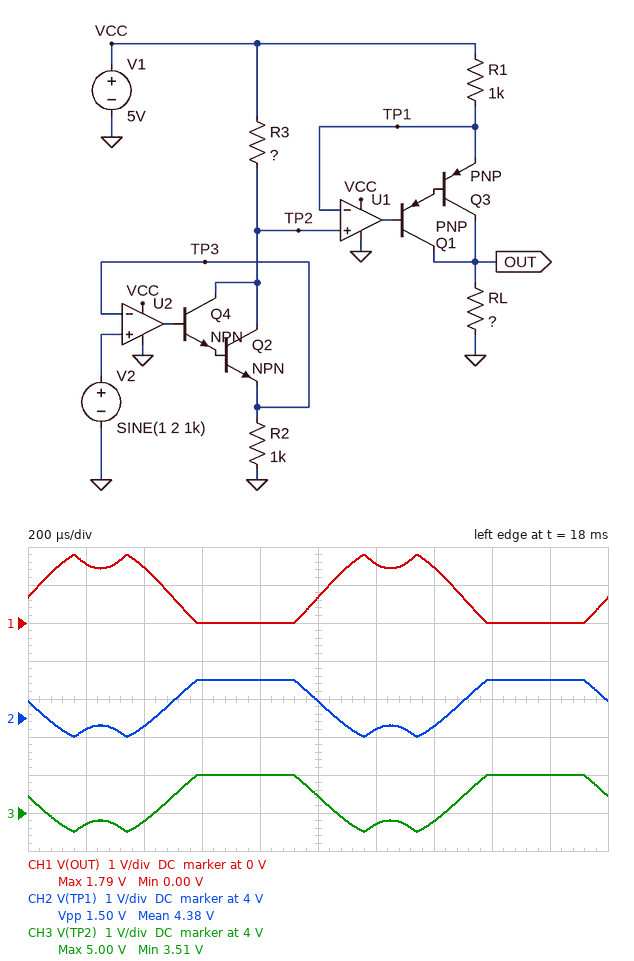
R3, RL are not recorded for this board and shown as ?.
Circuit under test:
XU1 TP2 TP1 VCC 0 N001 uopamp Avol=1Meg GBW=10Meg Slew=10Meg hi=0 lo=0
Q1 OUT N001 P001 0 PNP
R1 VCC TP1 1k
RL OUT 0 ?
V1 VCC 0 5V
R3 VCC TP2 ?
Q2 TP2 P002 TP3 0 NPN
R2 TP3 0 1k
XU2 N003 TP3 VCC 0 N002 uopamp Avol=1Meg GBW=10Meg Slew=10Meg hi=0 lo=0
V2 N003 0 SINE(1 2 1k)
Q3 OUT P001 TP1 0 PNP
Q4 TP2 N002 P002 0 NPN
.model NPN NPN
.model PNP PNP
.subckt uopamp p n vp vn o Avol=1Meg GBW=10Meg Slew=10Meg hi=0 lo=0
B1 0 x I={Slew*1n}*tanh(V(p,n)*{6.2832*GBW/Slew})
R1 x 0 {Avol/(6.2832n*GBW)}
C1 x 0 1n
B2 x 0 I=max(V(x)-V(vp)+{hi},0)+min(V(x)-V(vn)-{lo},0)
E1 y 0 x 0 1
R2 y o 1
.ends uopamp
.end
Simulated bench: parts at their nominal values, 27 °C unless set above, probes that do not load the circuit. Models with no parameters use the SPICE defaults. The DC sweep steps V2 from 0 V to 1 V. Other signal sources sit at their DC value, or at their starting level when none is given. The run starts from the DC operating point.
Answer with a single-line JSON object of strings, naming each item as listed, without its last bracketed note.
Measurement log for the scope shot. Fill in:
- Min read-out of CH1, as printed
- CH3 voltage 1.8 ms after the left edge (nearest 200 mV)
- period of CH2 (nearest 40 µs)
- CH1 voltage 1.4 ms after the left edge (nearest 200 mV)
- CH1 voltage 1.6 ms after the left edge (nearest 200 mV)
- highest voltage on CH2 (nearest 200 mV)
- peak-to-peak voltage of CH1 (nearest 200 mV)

{"Min read-out of CH1, as printed": "0.00 V", "CH3 voltage 1.8 ms after the left edge": "5.0 V", "period of CH2": "1.00 ms", "CH1 voltage 1.4 ms after the left edge": "1.4 V", "CH1 voltage 1.6 ms after the left edge": "0 V", "highest voltage on CH2": "5.0 V", "peak-to-peak voltage of CH1": "1.8 V"}
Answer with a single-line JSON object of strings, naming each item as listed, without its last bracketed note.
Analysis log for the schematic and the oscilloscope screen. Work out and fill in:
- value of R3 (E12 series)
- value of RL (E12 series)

{"value of R3": "560 Ω", "value of RL": "1.2 kΩ"}
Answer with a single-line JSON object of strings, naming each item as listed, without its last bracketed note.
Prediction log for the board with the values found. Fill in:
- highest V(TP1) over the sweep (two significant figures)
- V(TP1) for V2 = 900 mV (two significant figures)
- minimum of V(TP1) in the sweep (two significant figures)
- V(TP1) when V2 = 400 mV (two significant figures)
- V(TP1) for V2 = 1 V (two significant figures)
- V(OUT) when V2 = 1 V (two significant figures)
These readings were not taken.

{"highest V(TP1) over the sweep": "5.0 V", "V(TP1) for V2 = 900 mV": "4.5 V", "minimum of V(TP1) in the sweep": "4.4 V", "V(TP1) when V2 = 400 mV": "4.8 V", "V(TP1) for V2 = 1 V": "4.4 V", "V(OUT) when V2 = 1 V": "670 mV"}
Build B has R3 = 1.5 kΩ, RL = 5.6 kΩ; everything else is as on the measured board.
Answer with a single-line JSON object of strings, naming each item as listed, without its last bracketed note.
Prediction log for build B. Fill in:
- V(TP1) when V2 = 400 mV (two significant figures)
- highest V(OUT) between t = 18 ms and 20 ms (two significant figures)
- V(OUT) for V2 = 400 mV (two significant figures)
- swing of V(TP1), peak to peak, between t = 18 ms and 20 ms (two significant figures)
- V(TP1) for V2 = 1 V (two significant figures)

{"V(TP1) when V2 = 400 mV": "4.4 V", "highest V(OUT) between t = 18 ms and 20 ms": "3.6 V", "V(OUT) for V2 = 400 mV": "3.4 V", "swing of V(TP1), peak to peak, between t = 18 ms and 20 ms": "2.5 V", "V(TP1) for V2 = 1 V": "3.5 V"}
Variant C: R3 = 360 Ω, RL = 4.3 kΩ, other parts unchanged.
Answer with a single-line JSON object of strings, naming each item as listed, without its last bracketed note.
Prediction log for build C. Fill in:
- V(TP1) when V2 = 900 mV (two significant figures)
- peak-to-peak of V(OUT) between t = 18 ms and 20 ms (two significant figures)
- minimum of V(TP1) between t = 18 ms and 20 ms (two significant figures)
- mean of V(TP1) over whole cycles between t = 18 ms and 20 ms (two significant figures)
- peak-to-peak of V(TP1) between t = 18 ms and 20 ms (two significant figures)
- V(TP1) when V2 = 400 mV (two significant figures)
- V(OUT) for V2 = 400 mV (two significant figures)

{"V(TP1) when V2 = 900 mV": "4.7 V", "peak-to-peak of V(OUT) between t = 18 ms and 20 ms": "3.4 V", "minimum of V(TP1) between t = 18 ms and 20 ms": "3.9 V", "mean of V(TP1) over whole cycles between t = 18 ms and 20 ms": "4.6 V", "peak-to-peak of V(TP1) between t = 18 ms and 20 ms": "1.1 V", "V(TP1) when V2 = 400 mV": "4.9 V", "V(OUT) for V2 = 400 mV": "620 mV"}
